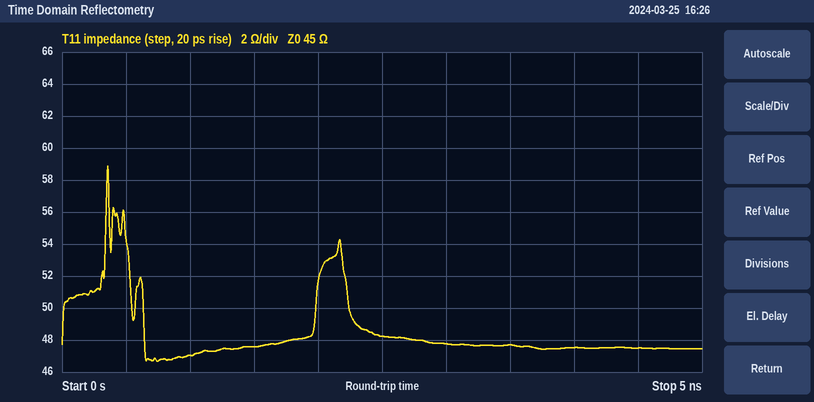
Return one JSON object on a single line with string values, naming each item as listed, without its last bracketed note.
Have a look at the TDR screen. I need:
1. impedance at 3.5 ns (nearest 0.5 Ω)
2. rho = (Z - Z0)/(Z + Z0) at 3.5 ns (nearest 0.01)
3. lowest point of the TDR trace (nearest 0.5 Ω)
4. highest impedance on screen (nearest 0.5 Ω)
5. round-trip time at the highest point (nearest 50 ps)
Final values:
{"impedance at 3.5 ns": "47.5 Ω", "rho = (Z - Z0)/(Z + Z0) at 3.5 ns": "+0.03", "lowest point of the TDR trace": "46.5 Ω", "highest impedance on screen": "59.0 Ω", "round-trip time at the highest point": "350 ps"}
